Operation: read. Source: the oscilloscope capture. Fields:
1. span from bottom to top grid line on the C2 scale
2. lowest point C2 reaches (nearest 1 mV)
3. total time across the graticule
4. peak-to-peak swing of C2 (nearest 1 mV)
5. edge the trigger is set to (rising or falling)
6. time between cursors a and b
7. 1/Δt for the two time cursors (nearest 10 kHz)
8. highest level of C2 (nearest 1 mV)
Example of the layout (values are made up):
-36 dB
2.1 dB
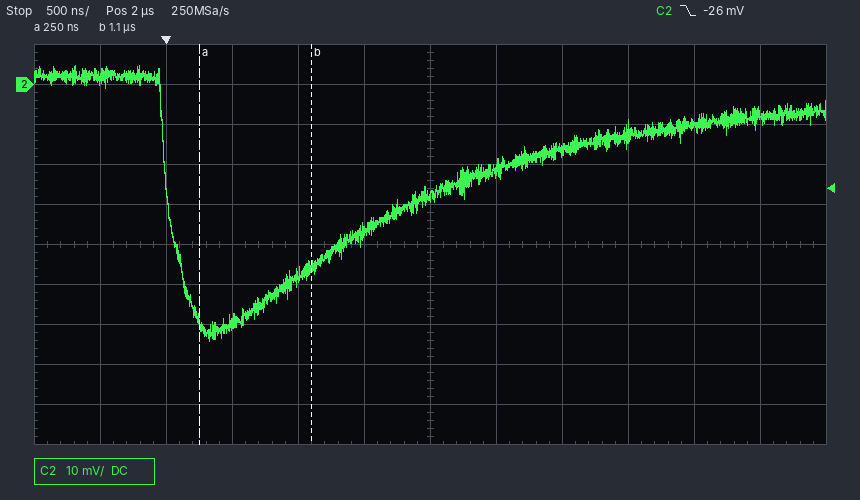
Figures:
100 mV
-64 mV
6 µs
69 mV
falling
850 ns
1.18 MHz
5 mV
